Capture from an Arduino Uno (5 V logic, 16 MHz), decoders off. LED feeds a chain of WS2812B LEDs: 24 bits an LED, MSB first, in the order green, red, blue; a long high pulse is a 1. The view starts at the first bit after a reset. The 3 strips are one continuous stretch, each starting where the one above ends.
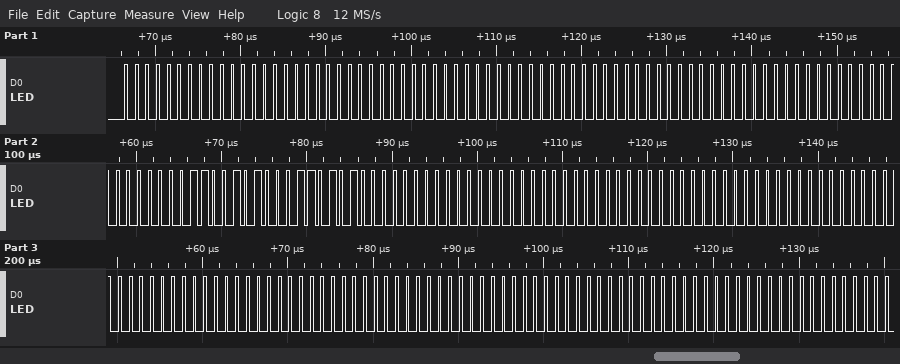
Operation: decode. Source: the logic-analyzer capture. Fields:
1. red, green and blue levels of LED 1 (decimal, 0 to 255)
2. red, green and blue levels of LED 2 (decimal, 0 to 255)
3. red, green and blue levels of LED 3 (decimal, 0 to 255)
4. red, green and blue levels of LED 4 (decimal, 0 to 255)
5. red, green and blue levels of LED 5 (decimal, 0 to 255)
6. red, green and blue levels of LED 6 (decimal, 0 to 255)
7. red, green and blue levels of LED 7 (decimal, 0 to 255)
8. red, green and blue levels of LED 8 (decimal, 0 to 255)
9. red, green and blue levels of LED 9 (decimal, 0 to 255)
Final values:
0, 0, 0
0, 0, 0
0, 0, 0
202, 0, 53
0, 0, 0
0, 0, 0
0, 0, 0
0, 0, 0
0, 0, 0
